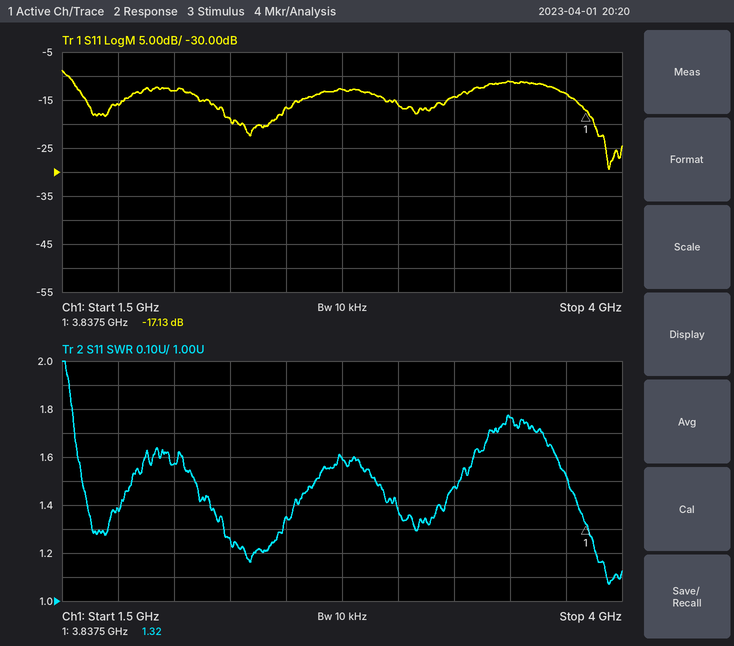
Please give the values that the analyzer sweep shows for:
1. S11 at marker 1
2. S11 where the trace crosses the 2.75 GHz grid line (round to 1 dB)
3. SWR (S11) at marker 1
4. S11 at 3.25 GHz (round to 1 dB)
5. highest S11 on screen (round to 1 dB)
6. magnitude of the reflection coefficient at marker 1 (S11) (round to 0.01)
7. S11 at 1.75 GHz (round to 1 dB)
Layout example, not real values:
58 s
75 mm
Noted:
-17.13 dB
-13 dB
1.32
-14 dB
-9 dB
0.14
-16 dB
